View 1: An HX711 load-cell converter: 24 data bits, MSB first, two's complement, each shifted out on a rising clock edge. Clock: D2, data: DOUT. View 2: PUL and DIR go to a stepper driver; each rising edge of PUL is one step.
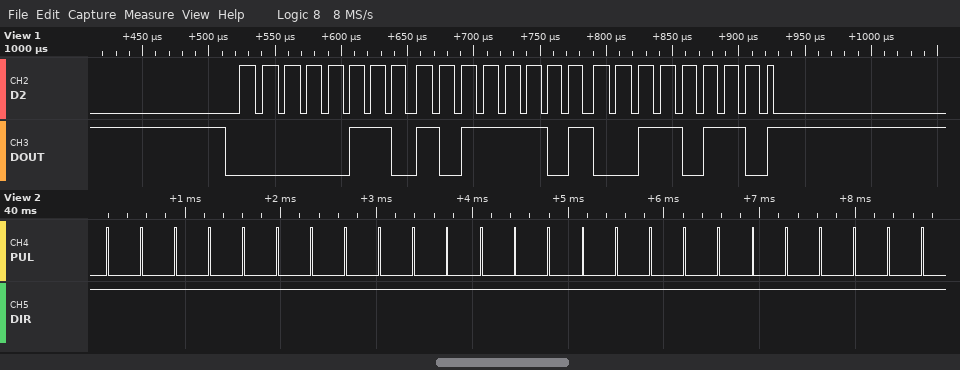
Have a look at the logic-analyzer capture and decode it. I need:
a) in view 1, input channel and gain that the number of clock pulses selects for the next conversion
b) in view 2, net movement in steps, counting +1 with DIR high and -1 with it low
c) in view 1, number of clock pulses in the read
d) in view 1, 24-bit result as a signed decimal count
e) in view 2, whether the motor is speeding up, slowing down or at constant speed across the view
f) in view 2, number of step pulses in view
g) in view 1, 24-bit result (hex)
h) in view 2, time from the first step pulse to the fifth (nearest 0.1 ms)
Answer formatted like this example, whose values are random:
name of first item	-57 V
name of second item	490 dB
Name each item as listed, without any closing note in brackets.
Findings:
in view 1, input channel and gain that the number of clock pulses selects for the next conversion	channel A, gain 128
in view 2, net movement in steps, counting +1 with DIR high and -1 with it low	+25
in view 1, number of clock pulses in the read	25
in view 1, 24-bit result as a signed decimal count	441654
in view 2, whether the motor is speeding up, slowing down or at constant speed across the view	constant speed
in view 2, number of step pulses in view	25
in view 1, 24-bit result	0x06BD36
in view 2, time from the first step pulse to the fifth	1.4 ms
